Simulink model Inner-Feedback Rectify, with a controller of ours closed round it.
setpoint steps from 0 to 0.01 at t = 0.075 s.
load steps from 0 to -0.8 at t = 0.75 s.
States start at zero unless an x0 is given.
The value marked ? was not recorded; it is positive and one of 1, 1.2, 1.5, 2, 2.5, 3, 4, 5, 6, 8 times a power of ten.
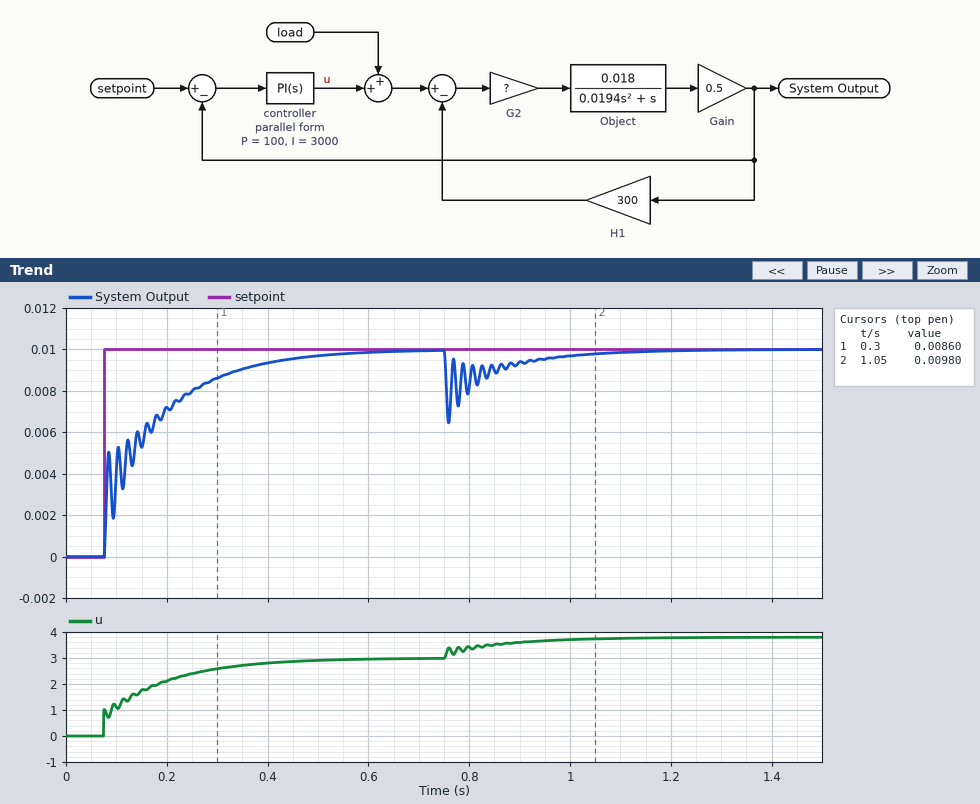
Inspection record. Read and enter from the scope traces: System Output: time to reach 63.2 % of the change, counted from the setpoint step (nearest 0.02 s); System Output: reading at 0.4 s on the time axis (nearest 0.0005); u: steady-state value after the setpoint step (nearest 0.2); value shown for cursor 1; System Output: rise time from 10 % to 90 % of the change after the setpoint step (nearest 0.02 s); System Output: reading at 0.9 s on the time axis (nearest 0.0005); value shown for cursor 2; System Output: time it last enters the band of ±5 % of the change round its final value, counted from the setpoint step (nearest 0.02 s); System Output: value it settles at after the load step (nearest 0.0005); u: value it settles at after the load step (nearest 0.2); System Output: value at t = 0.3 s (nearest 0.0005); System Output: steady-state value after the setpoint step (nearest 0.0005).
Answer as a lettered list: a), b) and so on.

a) 0.08 s
b) 0.0095
c) 3.0
d) 0.00860
e) 0.26 s
f) 0.0095
g) 0.00980
h) 0.36 s
i) 0.0100
j) 3.8
k) 0.0085
l) 0.0100
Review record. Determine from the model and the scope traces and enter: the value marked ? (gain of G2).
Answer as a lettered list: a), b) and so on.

a) 600
